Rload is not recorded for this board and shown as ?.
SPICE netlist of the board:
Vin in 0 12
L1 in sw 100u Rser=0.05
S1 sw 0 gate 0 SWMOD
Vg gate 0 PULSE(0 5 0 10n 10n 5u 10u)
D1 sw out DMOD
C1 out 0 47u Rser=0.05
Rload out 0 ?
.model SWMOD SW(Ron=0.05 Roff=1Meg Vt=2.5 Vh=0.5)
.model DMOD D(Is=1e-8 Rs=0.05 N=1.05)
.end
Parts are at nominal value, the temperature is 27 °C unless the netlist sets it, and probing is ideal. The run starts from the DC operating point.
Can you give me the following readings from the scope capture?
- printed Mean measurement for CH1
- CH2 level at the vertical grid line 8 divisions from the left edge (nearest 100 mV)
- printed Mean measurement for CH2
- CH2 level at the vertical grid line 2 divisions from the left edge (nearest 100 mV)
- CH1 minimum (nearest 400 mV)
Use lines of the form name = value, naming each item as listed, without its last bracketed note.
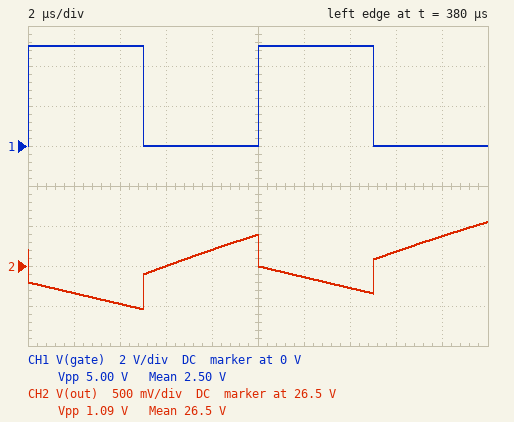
printed Mean measurement for CH1 = 2.50 V
CH2 level at the vertical grid line 8 divisions from the left edge = 26.7 V
printed Mean measurement for CH2 = 26.5 V
CH2 level at the vertical grid line 2 divisions from the left edge = 26.0 V
CH1 minimum = 0 V
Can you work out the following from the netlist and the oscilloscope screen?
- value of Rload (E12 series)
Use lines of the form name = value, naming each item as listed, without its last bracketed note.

value of Rload = 8.2 Ω
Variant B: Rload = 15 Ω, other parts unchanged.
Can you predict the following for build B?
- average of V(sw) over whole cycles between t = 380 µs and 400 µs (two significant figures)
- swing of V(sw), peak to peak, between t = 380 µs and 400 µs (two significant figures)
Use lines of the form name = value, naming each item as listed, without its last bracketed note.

average of V(sw) over whole cycles between t = 380 µs and 400 µs = 15 V
swing of V(sw), peak to peak, between t = 380 µs and 400 µs = 30 V
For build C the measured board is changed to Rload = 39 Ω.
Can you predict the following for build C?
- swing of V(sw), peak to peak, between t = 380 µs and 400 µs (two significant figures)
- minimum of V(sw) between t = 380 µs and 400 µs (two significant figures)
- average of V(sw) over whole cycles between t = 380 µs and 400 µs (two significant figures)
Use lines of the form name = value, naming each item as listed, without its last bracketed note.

swing of V(sw), peak to peak, between t = 380 µs and 400 µs = 32 V
minimum of V(sw) between t = 380 µs and 400 µs = 150 mV
average of V(sw) over whole cycles between t = 380 µs and 400 µs = 16 V
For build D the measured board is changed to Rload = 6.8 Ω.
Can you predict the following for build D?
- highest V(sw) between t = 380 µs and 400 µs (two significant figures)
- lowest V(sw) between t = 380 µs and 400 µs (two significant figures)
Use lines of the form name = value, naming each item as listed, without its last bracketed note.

highest V(sw) between t = 380 µs and 400 µs = 27 V
lowest V(sw) between t = 380 µs and 400 µs = 450 mV
